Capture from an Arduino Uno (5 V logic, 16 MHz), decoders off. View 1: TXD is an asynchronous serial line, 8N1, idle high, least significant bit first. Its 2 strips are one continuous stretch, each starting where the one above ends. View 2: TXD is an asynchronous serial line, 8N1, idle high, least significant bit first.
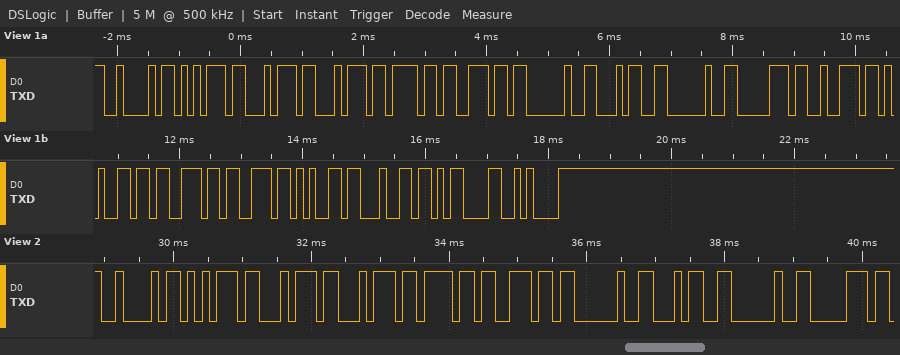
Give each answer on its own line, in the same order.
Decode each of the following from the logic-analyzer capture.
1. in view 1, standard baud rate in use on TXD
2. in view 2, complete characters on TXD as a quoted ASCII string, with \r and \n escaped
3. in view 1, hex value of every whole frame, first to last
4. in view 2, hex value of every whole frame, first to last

9600 baud
"Button 4 p"
42 75 74 74 6F 6E 20 34 20 70 72 65 73 73 65 64 0D 0A
42 75 74 74 6F 6E 20 34 20 70
